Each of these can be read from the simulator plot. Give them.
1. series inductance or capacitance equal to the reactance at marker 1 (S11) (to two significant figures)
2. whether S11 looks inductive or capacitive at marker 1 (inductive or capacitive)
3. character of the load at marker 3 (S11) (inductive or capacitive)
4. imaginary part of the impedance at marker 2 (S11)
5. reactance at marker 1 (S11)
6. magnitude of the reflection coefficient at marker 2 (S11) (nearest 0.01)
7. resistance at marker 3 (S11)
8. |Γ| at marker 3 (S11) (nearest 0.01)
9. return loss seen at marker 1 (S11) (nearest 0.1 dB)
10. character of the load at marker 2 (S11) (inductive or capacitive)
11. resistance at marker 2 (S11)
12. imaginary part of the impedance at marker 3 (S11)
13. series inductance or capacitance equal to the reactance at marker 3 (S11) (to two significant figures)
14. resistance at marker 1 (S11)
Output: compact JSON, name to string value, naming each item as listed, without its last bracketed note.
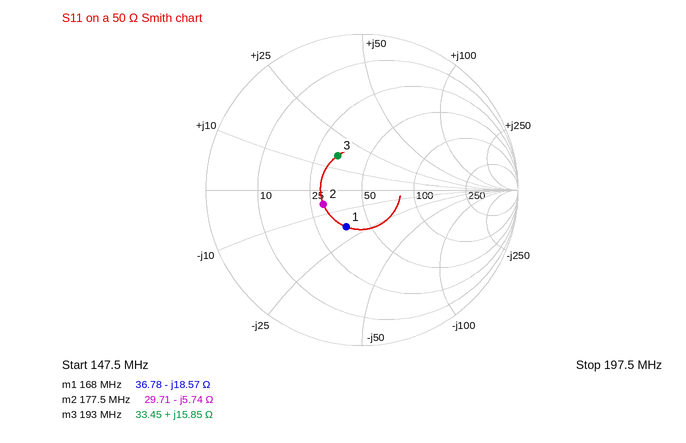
{"series inductance or capacitance equal to the reactance at marker 1 (S11)": "51 pF", "whether S11 looks inductive or capacitive at marker 1": "capacitive", "character of the load at marker 3 (S11)": "inductive", "imaginary part of the impedance at marker 2": "-5.74 Ω", "reactance at marker 1": "-18.57 Ω", "magnitude of the reflection coefficient at marker 2 (S11)": "0.26", "resistance at marker 3": "33.45 Ω", "|Γ| at marker 3 (S11)": "0.27", "return loss seen at marker 1 (S11)": "11.8 dB", "character of the load at marker 2 (S11)": "capacitive", "resistance at marker 2": "29.71 Ω", "imaginary part of the impedance at marker 3": "+15.85 Ω", "series inductance or capacitance equal to the reactance at marker 3 (S11)": "13 nH", "resistance at marker 1": "36.78 Ω"}
